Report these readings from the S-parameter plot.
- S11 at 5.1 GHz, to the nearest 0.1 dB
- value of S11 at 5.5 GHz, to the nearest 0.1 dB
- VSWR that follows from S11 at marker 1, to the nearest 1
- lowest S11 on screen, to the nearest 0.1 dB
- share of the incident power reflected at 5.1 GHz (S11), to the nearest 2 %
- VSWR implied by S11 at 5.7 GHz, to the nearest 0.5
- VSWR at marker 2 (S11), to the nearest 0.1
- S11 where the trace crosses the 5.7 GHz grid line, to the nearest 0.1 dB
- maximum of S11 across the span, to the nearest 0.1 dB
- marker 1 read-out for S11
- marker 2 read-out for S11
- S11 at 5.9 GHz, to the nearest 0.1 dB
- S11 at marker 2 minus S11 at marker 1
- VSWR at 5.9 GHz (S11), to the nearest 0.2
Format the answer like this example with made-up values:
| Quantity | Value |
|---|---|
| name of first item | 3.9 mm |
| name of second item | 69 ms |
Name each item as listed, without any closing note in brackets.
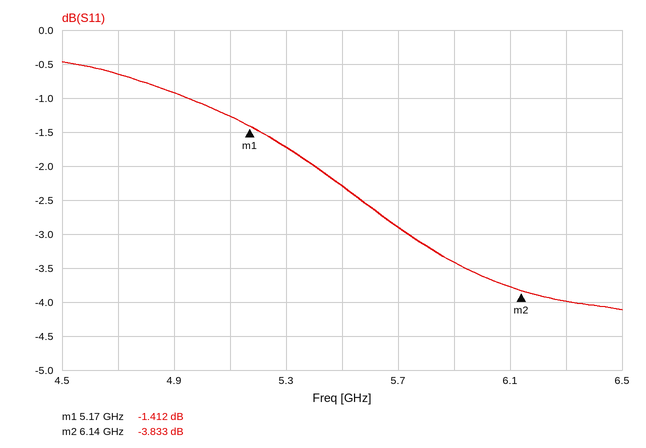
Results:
| Quantity | Value |
|---|---|
| S11 at 5.1 GHz, to the nearest 0.1 dB | -1.3 dB |
| value of S11 at 5.5 GHz, to the nearest 0.1 dB | -2.3 dB |
| VSWR that follows from S11 at marker 1, to the nearest 1 | 12 |
| lowest S11 on screen, to the nearest 0.1 dB | -4.1 dB |
| share of the incident power reflected at 5.1 GHz (S11), to the nearest 2 % | 74 % |
| VSWR implied by S11 at 5.7 GHz, to the nearest 0.5 | 6.0 |
| VSWR at marker 2 (S11), to the nearest 0.1 | 4.6 |
| S11 where the trace crosses the 5.7 GHz grid line, to the nearest 0.1 dB | -2.9 dB |
| maximum of S11 across the span, to the nearest 0.1 dB | -0.5 dB |
| marker 1 read-out for S11 | -1.412 dB |
| marker 2 read-out for S11 | -3.833 dB |
| S11 at 5.9 GHz, to the nearest 0.1 dB | -3.4 dB |
| S11 at marker 2 minus S11 at marker 1 | -2.421 dB |
| VSWR at 5.9 GHz (S11), to the nearest 0.2 | 5.2 |
